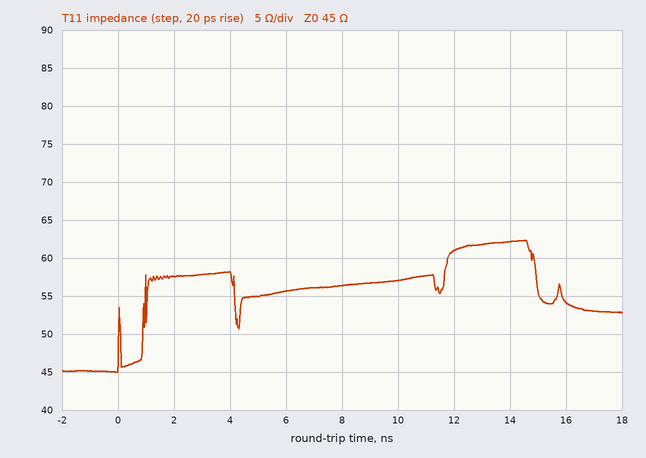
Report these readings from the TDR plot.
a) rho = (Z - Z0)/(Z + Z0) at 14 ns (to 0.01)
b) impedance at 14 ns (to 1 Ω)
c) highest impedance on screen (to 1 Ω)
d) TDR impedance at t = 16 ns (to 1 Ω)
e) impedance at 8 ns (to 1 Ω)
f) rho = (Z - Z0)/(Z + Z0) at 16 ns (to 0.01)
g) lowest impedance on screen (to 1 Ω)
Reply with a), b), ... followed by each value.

a) +0.16
b) 62 Ω
c) 62 Ω
d) 54 Ω
e) 56 Ω
f) +0.09
g) 45 Ω
